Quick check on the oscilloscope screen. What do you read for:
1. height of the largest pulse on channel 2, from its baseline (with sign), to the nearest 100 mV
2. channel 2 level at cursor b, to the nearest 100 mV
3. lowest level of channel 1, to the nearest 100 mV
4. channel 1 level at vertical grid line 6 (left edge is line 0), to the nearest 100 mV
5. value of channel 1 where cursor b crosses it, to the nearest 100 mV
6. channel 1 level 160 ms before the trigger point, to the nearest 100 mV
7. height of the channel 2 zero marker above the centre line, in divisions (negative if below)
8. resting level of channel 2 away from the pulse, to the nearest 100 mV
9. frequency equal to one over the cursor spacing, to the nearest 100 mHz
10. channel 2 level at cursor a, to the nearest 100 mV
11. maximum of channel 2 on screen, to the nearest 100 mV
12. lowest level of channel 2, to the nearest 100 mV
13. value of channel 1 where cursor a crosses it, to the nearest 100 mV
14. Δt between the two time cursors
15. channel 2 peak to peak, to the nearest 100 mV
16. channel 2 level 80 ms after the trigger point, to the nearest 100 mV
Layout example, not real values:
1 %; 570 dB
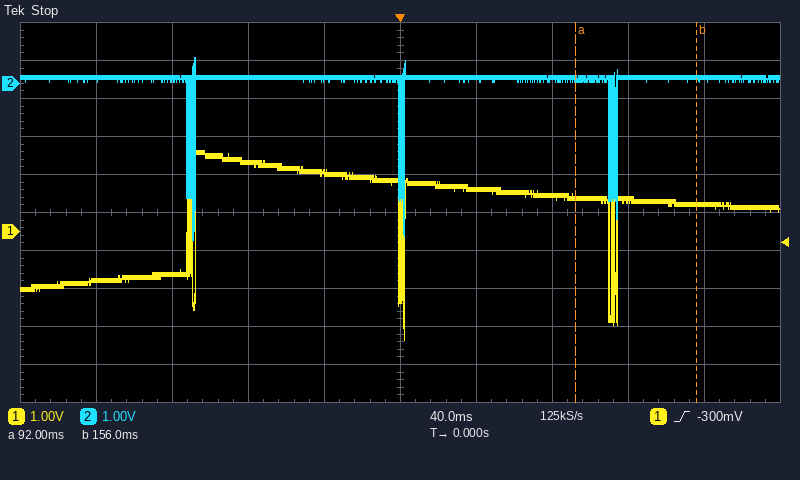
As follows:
-4.3 V; 100 mV; -2.8 V; 1.1 V; 700 mV; -1.3 V; +3.4 div; 200 mV; 15.6 Hz; 100 mV; 700 mV; -4.1 V; 900 mV; 64 ms; 4.8 V; 100 mV
